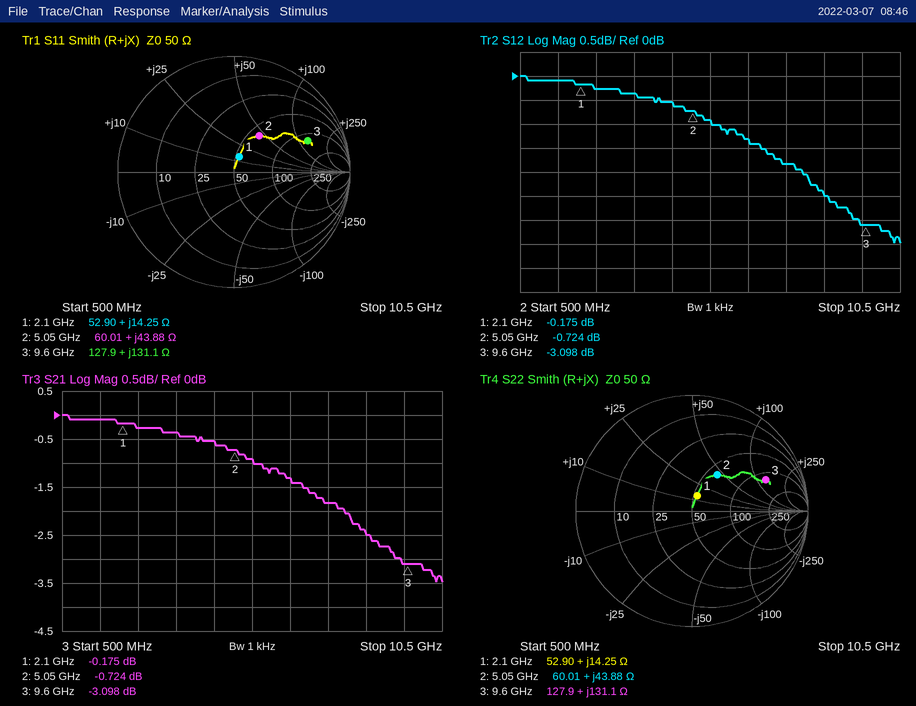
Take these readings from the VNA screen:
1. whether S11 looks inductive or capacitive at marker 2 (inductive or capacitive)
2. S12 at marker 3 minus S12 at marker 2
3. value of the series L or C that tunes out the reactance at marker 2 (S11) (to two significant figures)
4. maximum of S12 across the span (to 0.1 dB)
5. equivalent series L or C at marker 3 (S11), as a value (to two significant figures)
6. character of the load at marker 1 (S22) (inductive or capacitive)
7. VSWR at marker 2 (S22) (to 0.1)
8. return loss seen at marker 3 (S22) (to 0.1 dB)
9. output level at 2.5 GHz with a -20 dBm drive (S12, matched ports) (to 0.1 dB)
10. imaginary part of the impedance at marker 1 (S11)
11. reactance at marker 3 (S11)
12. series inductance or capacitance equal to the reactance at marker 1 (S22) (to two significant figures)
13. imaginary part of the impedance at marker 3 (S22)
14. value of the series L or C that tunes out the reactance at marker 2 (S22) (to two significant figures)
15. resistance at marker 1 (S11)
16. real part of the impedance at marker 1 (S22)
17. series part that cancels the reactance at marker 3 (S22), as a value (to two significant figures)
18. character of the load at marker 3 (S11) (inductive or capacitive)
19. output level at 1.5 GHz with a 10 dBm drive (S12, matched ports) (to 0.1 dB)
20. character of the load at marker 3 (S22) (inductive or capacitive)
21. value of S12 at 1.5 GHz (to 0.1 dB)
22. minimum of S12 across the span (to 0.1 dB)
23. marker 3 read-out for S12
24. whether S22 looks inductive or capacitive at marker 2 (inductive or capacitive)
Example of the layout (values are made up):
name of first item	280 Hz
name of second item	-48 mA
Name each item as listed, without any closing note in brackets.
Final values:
whether S11 looks inductive or capacitive at marker 2	inductive
S12 at marker 3 minus S12 at marker 2	-2.374 dB
value of the series L or C that tunes out the reactance at marker 2 (S11)	720 fF
maximum of S12 across the span	0.0 dB
equivalent series L or C at marker 3 (S11), as a value	2.2 nH
character of the load at marker 1 (S22)	inductive
VSWR at marker 2 (S22)	2.2
return loss seen at marker 3 (S22)	3.2 dB
output level at 2.5 GHz with a -20 dBm drive (S12, matched ports)	-20.3 dBm
imaginary part of the impedance at marker 1	+14.25 Ω
reactance at marker 3	+131.1 Ω
series inductance or capacitance equal to the reactance at marker 1 (S22)	1.1 nH
imaginary part of the impedance at marker 3	+131.1 Ω
value of the series L or C that tunes out the reactance at marker 2 (S22)	720 fF
resistance at marker 1	52.90 Ω
real part of the impedance at marker 1	52.90 Ω
series part that cancels the reactance at marker 3 (S22), as a value	130 fF
character of the load at marker 3 (S11)	inductive
output level at 1.5 GHz with a 10 dBm drive (S12, matched ports)	9.9 dBm
character of the load at marker 3 (S22)	inductive
value of S12 at 1.5 GHz	-0.1 dB
minimum of S12 across the span	-3.5 dB
marker 3 read-out for S12	-3.098 dB
whether S22 looks inductive or capacitive at marker 2	inductive
